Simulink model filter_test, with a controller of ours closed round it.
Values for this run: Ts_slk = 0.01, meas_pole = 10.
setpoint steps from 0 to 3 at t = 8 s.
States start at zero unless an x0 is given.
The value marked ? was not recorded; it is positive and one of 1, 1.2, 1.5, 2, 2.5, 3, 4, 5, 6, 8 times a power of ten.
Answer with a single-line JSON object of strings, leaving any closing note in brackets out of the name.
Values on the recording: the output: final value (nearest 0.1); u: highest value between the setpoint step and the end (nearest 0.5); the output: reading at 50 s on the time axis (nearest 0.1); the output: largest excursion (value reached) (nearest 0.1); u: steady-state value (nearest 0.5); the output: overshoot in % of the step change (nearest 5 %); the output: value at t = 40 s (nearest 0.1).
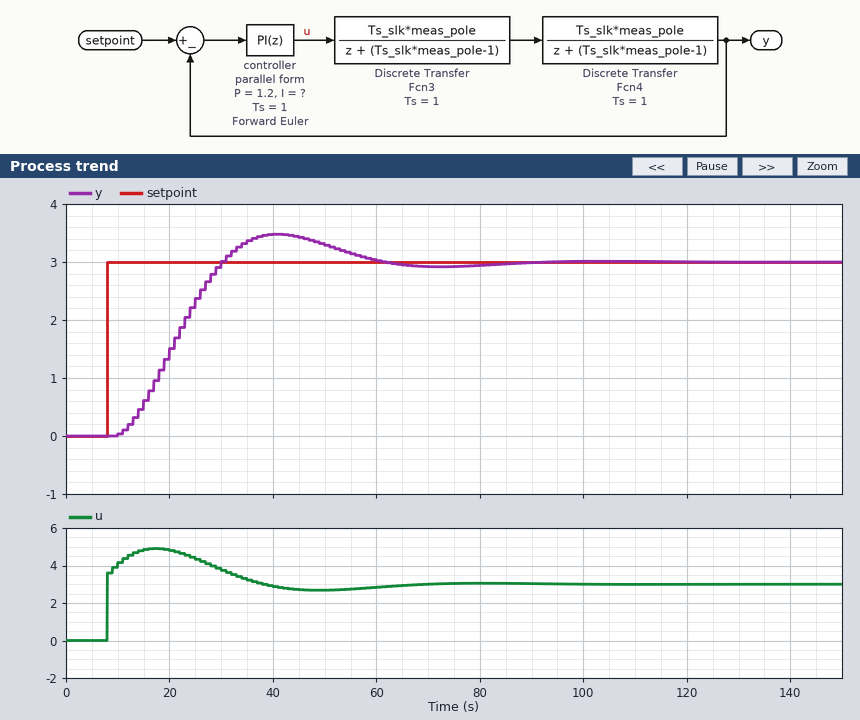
{"the output: final value": "3.0", "u: highest value between the setpoint step and the end": "5.0", "the output: reading at 50 s on the time axis": "3.3", "the output: largest excursion (value reached)": "3.5", "u: steady-state value": "3.0", "the output: overshoot in % of the step change": "15 %", "the output: value at t = 40 s": "3.5"}
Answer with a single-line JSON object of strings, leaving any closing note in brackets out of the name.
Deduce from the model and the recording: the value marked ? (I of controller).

{"the value marked ?": "0.1"}
